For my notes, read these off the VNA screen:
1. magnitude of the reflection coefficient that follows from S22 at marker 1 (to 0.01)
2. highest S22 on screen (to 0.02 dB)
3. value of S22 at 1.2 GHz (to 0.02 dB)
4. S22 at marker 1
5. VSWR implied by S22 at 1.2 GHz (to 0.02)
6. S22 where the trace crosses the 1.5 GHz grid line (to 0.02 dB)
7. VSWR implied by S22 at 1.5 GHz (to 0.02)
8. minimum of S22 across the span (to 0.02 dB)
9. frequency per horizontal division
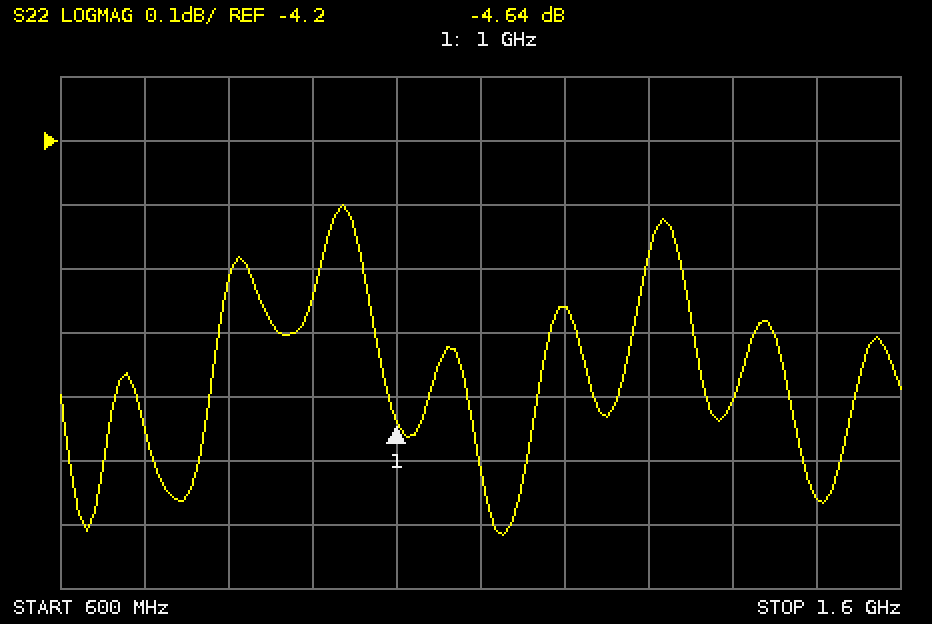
0.59
-4.30 dB
-4.46 dB
-4.64 dB
3.98
-4.76 dB
3.74
-4.82 dB
100 MHz
